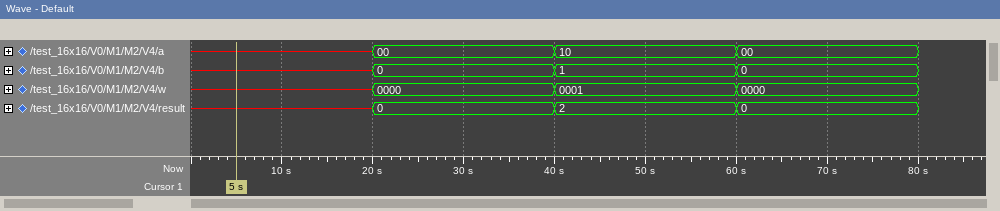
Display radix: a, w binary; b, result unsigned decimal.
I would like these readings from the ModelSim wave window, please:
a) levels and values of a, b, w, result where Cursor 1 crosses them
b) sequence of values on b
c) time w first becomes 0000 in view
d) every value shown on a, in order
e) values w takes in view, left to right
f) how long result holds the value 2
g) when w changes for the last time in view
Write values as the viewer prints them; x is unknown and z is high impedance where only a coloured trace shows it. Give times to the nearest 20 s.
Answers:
a=x, b=x, w=x, result=x
x, 0, 1, 0
20 s
x, 00, 10, 00
x, 0000, 0001, 0000
20 s
60 s
